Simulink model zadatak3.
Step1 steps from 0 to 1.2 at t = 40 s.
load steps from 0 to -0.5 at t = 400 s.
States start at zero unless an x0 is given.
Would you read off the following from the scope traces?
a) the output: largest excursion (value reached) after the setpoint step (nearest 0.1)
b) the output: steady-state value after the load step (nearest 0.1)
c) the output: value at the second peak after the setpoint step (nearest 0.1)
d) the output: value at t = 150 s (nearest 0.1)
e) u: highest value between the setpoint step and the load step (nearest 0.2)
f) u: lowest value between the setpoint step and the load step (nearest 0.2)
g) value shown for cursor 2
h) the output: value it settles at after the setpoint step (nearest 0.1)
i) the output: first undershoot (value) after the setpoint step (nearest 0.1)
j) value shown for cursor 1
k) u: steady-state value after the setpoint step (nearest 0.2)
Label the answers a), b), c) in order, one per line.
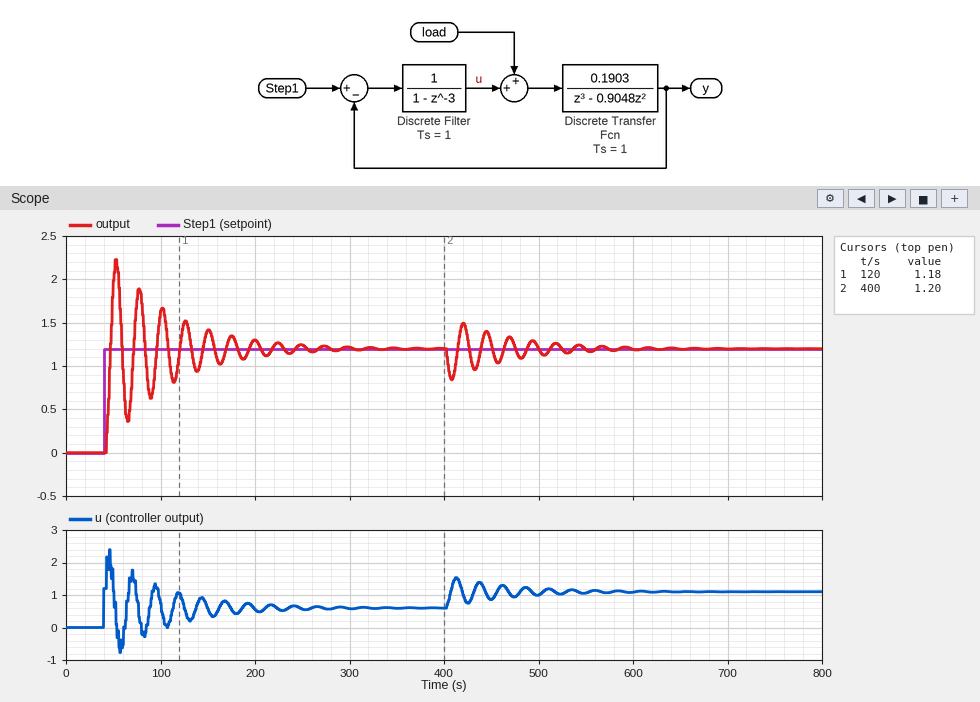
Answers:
a) 2.2
b) 1.2
c) 1.9
d) 1.4
e) 2.4
f) -0.8
g) 1.20
h) 1.2
i) 0.4
j) 1.18
k) 0.6
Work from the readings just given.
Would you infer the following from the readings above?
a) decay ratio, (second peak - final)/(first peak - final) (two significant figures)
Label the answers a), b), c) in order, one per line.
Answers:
a) 0.70
